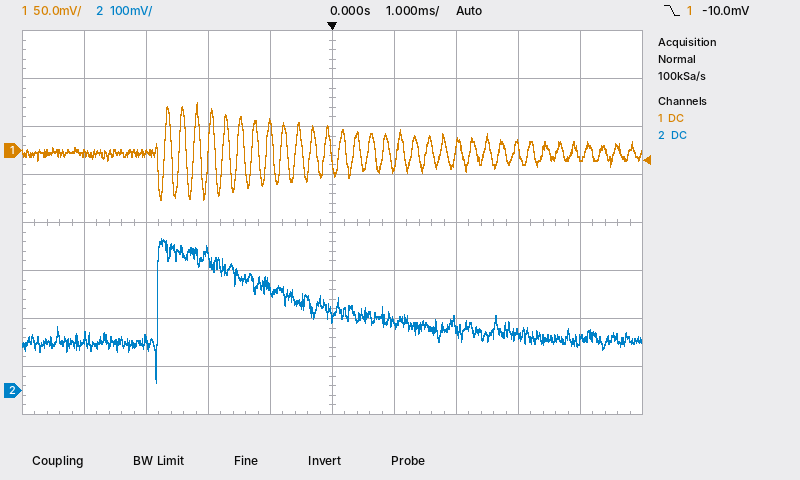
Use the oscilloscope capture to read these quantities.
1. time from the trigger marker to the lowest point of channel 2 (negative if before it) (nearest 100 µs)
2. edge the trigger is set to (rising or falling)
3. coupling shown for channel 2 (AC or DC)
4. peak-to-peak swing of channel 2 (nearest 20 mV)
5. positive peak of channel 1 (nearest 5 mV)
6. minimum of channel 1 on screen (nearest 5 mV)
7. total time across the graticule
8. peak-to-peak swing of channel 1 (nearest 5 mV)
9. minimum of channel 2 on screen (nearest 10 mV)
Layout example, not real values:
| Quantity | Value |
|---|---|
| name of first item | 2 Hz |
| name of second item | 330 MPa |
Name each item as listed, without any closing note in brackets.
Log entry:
| Quantity | Value |
|---|---|
| time from the trigger marker to the lowest point of channel 2 (negative if before it) | -2.8 ms |
| edge the trigger is set to | falling |
| coupling shown for channel 2 | DC |
| peak-to-peak swing of channel 2 | 300 mV |
| positive peak of channel 1 | 50 mV |
| minimum of channel 1 on screen | -50 mV |
| total time across the graticule | 10 ms |
| peak-to-peak swing of channel 1 | 100 mV |
| minimum of channel 2 on screen | 20 mV |
